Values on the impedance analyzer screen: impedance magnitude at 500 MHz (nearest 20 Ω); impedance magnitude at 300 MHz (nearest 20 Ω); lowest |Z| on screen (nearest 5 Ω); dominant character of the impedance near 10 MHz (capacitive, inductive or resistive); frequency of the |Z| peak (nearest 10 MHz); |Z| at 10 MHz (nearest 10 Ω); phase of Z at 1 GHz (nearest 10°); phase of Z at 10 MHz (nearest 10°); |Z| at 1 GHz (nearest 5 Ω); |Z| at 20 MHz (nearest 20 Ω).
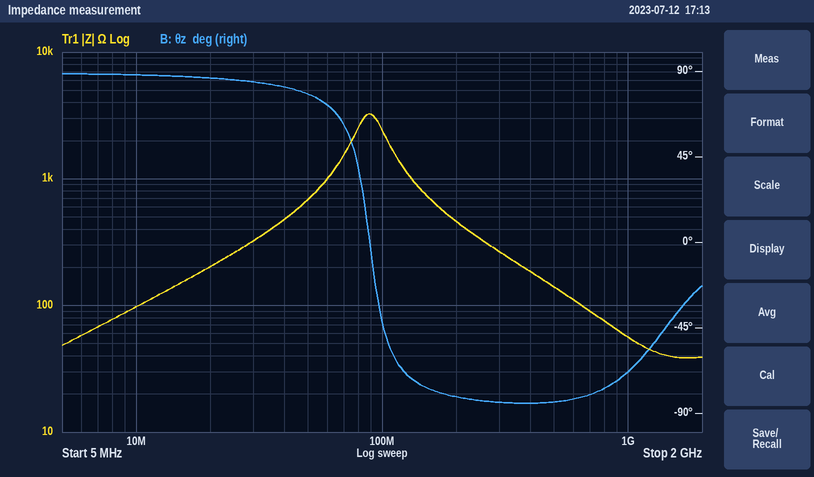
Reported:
140 Ω
260 Ω
40 Ω
inductive
90 MHz
100 Ω
-70°
90°
55 Ω
200 Ω
